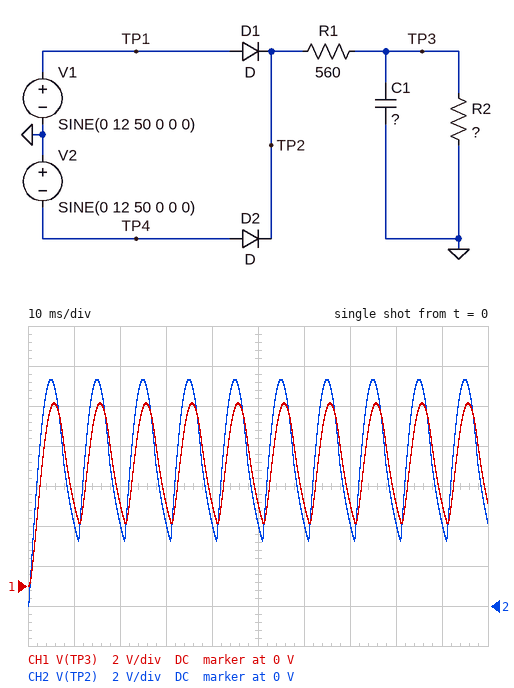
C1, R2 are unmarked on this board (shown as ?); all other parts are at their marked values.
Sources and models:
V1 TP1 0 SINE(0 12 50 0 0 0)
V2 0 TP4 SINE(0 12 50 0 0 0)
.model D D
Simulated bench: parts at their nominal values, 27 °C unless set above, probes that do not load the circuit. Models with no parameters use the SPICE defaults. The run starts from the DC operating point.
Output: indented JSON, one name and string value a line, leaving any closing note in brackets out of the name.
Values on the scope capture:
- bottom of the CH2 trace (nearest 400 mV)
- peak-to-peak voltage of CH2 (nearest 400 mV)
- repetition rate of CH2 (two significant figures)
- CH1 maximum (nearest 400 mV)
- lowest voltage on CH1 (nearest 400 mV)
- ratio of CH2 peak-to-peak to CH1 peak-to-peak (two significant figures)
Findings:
{
  "bottom of the CH2 trace": "0 V",
  "peak-to-peak voltage of CH2": "11.2 V",
  "repetition rate of CH2": "100 Hz",
  "CH1 maximum": "9.2 V",
  "lowest voltage on CH1": "0 V",
  "ratio of CH2 peak-to-peak to CH1 peak-to-peak": "1.2"
}
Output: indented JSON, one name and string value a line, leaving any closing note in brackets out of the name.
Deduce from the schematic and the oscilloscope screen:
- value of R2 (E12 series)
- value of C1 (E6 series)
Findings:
{
  "value of R2": "2.7 kΩ",
  "value of C1": "1.5 µF"
}
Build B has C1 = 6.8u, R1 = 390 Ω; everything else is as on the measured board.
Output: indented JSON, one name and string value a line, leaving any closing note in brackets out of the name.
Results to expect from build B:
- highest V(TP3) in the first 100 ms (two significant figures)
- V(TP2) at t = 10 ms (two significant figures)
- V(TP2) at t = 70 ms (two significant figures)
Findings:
{
  "highest V(TP3) in the first 100 ms": "8.8 V",
  "V(TP2) at t = 10 ms": "7.0 V",
  "V(TP2) at t = 70 ms": "7.4 V"
}
